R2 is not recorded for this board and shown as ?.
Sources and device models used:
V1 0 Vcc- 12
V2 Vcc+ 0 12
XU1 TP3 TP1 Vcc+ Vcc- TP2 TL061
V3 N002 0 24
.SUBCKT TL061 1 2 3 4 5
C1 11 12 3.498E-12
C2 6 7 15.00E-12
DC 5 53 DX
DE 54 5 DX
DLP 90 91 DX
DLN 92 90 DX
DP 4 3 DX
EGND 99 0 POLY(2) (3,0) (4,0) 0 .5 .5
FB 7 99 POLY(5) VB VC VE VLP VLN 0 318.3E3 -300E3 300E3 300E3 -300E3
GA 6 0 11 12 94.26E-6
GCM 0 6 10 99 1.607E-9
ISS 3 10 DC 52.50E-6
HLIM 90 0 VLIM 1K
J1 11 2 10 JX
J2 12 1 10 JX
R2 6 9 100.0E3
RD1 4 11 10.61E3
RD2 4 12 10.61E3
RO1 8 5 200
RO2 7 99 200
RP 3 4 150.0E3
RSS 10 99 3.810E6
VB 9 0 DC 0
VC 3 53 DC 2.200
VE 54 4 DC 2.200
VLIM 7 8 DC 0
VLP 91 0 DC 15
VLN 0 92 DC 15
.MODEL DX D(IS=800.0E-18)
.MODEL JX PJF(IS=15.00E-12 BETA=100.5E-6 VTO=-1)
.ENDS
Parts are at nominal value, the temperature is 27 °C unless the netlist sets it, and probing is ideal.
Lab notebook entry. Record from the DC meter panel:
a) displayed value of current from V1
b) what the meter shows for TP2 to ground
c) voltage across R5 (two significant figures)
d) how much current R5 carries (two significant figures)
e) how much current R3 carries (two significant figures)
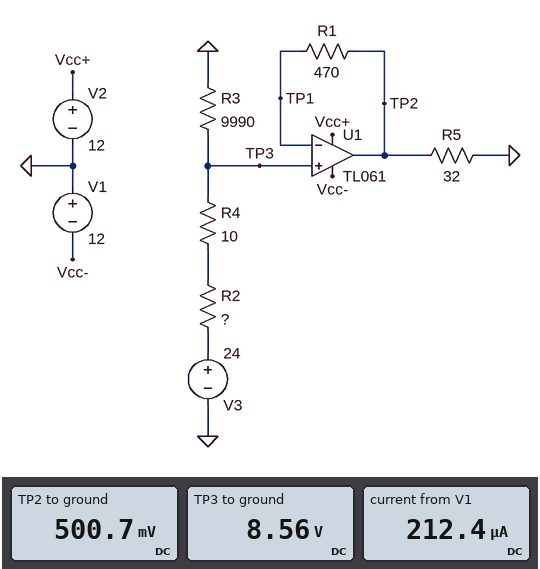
212.4 µA
500.7 mV
500 mV
16 mA
860 µA
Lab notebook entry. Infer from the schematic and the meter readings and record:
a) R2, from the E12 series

18 kΩ
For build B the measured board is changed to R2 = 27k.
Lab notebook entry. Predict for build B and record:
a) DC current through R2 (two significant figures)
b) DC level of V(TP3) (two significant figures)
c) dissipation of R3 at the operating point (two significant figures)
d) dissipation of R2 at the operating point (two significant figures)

650 µA
6.5 V
4.2 mW
11 mW
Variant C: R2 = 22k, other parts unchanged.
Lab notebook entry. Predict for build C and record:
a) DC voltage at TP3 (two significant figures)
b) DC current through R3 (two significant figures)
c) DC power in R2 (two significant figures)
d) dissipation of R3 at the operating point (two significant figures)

7.5 V
750 µA
12 mW
5.6 mW
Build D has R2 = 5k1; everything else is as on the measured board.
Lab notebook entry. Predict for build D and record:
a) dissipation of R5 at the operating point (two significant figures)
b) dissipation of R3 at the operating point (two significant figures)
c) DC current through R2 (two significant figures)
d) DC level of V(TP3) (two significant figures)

7.8 mW
25 mW
1.6 mA
16 V
